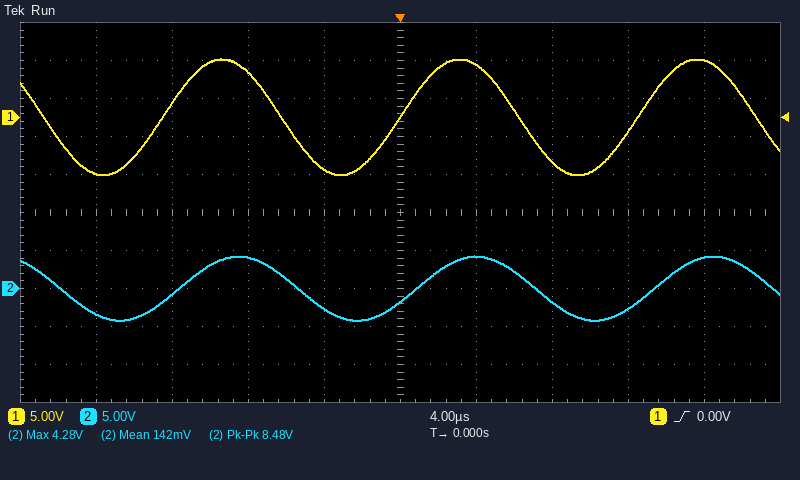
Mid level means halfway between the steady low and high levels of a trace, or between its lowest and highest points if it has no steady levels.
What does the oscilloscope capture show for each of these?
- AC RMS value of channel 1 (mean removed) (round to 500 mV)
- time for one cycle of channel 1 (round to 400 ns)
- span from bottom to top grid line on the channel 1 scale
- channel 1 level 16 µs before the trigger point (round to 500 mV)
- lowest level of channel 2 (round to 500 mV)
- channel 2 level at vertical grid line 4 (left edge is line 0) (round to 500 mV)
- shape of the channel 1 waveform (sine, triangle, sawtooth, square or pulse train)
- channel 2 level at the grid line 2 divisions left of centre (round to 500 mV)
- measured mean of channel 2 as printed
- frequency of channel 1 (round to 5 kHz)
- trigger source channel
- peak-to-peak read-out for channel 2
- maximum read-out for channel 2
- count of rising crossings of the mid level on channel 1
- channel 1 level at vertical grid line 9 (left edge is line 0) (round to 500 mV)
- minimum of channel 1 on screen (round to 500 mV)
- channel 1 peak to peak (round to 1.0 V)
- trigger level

5.5 V
12.4 µs
50 V
-7.5 V
-4.0 V
-2.5 V
sine
4.0 V
142 mV
80 kHz
channel 1
8.48 V
4.28 V
3
7.5 V
-7.5 V
15.0 V
0.00 V
